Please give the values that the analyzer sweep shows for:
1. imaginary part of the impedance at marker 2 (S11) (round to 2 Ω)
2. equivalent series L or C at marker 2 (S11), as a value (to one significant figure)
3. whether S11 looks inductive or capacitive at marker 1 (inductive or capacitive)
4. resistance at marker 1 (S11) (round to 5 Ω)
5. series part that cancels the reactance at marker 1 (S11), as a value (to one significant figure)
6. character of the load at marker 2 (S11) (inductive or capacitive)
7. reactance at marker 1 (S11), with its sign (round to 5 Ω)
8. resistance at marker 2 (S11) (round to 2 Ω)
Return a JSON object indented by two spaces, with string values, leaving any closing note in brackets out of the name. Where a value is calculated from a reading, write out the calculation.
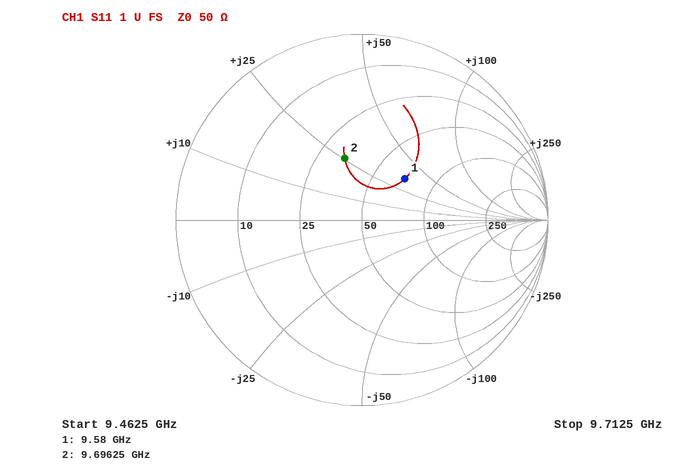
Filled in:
{
  "imaginary part of the impedance at marker 2 (S11)": "+26 Ω",
  "equivalent series L or C at marker 2 (S11), as a value": "L = 26 Ω/(2π × 9.69625 GHz) ≈ 427 pH, so 400 pH to one significant figure",
  "whether S11 looks inductive or capacitive at marker 1": "inductive",
  "resistance at marker 1 (S11)": "70 Ω",
  "series part that cancels the reactance at marker 1 (S11), as a value": "C = 1/(2π × 9.58 GHz × 35 Ω) ≈ 475 fF, so 500 fF to one significant figure",
  "character of the load at marker 2 (S11)": "inductive",
  "reactance at marker 1 (S11), with its sign": "+35 Ω",
  "resistance at marker 2 (S11)": "34 Ω"
}
